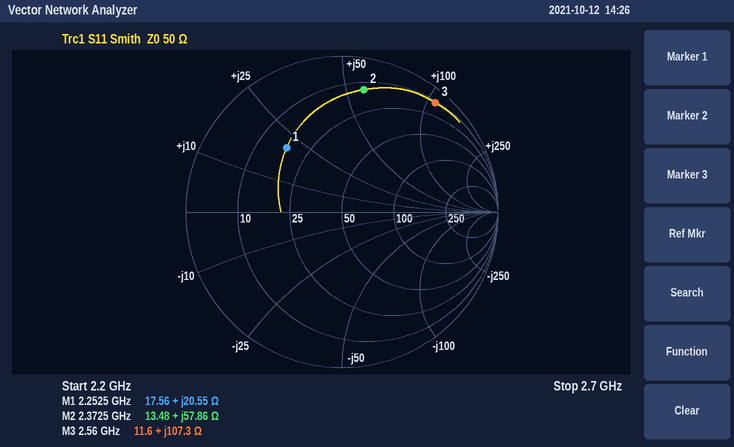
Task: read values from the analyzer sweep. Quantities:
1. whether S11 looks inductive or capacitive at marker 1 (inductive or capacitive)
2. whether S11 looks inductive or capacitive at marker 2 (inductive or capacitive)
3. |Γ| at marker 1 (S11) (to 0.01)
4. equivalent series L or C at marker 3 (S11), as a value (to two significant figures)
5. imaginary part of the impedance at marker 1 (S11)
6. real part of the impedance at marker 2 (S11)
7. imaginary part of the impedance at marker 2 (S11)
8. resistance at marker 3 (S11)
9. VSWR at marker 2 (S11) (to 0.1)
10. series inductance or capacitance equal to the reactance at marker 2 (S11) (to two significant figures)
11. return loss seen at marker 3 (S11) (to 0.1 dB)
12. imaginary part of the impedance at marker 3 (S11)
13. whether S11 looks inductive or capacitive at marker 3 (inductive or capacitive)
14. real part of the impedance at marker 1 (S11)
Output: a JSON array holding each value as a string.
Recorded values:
["inductive", "inductive", "0.54", "6.7 nH", "+20.55 Ω", "13.48 Ω", "+57.86 Ω", "11.6 Ω", "8.8", "3.9 nH", "0.7 dB", "+107.3 Ω", "inductive", "17.56 Ω"]
